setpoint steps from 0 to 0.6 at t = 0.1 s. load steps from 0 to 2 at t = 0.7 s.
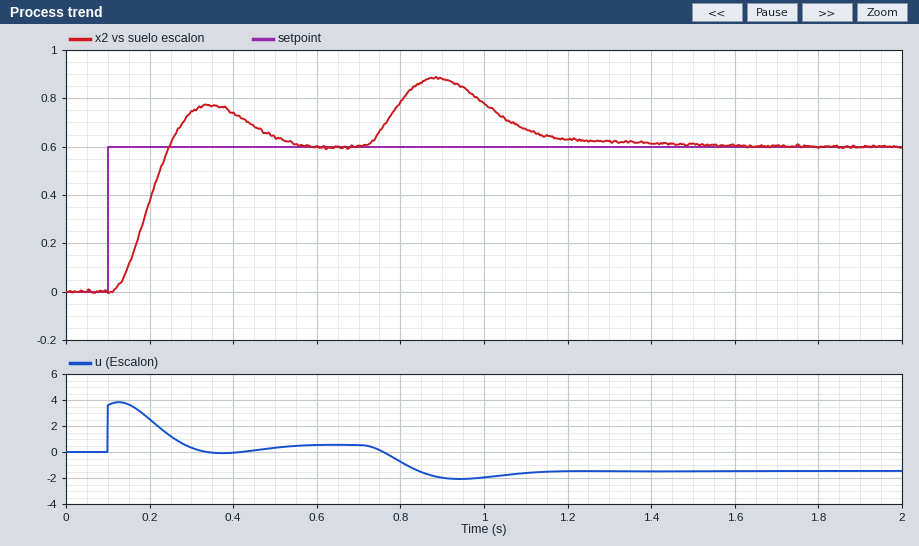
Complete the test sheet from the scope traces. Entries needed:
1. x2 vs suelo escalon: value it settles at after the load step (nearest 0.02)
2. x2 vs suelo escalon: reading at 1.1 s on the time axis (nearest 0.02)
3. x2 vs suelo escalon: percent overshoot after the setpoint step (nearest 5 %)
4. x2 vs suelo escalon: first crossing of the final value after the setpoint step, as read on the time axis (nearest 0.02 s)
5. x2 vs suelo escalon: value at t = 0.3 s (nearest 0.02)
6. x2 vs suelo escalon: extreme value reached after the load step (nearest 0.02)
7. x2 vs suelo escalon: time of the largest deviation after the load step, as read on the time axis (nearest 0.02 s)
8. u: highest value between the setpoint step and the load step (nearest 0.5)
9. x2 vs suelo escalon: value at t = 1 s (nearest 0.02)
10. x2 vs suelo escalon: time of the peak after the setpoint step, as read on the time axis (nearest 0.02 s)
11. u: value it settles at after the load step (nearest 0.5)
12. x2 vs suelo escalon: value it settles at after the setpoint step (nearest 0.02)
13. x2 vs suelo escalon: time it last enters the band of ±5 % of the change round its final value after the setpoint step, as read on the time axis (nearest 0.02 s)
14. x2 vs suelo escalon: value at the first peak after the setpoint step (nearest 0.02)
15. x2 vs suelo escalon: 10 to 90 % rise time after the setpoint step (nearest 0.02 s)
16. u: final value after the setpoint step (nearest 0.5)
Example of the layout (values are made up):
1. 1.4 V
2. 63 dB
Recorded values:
1. 0.60
2. 0.68
3. 30 %
4. 0.24 s
5. 0.74
6. 0.88
7. 0.88 s
8. 4.0
9. 0.78
10. 0.34 s
11. -1.5
12. 0.60
13. 0.52 s
14. 0.78
15. 0.10 s
16. 0.5
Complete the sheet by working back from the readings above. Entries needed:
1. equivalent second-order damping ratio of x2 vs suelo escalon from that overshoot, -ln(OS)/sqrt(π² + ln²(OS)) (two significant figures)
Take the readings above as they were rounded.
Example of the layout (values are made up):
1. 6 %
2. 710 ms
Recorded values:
1. 0.36
